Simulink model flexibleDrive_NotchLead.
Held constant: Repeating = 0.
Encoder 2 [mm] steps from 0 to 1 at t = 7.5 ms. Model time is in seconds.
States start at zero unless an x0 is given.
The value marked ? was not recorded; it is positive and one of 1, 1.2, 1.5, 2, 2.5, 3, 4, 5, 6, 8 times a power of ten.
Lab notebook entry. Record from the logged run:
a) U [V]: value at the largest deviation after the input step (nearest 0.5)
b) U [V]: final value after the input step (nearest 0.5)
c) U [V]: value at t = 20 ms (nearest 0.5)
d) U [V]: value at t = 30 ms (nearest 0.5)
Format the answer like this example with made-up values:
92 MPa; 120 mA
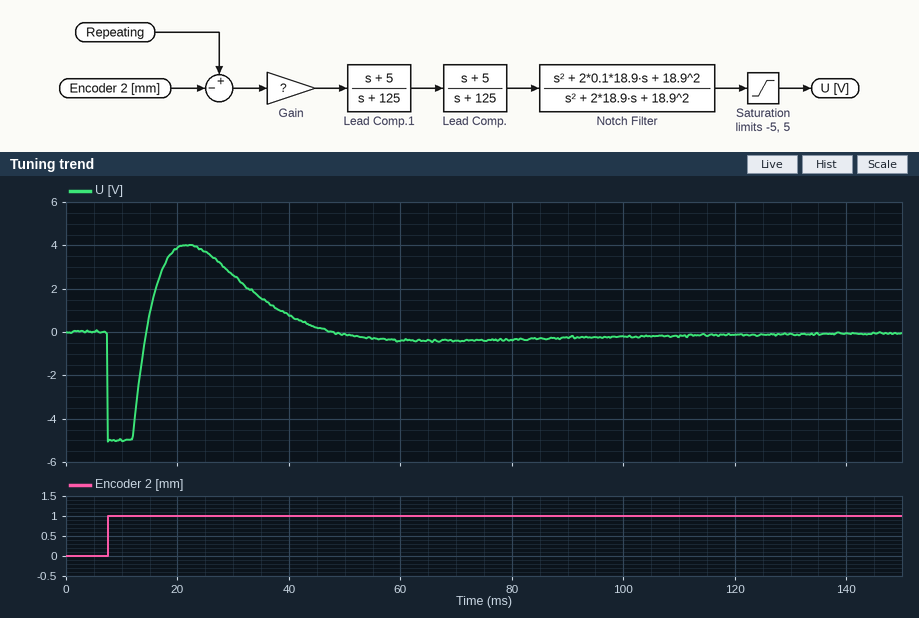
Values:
-5.0; 0.0; 4.0; 2.5
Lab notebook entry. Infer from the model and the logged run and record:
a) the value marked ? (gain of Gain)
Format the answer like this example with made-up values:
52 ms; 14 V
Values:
25
